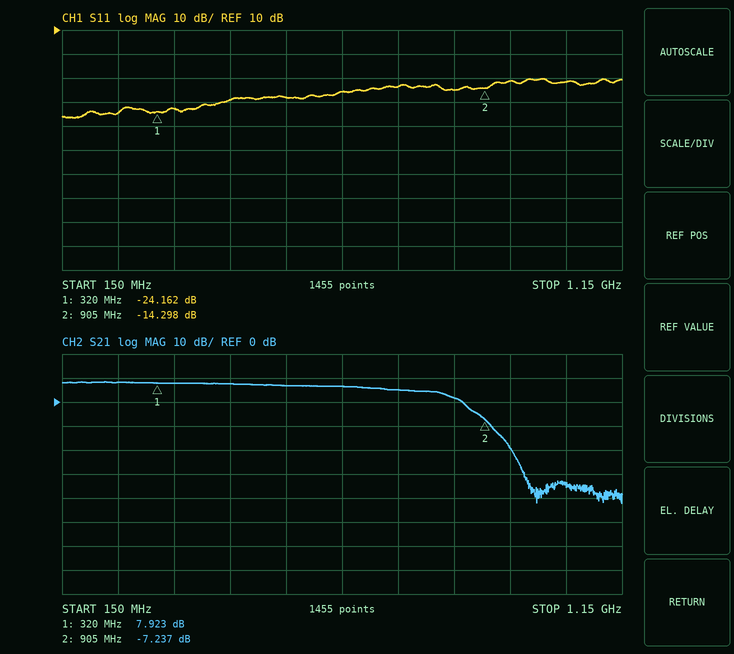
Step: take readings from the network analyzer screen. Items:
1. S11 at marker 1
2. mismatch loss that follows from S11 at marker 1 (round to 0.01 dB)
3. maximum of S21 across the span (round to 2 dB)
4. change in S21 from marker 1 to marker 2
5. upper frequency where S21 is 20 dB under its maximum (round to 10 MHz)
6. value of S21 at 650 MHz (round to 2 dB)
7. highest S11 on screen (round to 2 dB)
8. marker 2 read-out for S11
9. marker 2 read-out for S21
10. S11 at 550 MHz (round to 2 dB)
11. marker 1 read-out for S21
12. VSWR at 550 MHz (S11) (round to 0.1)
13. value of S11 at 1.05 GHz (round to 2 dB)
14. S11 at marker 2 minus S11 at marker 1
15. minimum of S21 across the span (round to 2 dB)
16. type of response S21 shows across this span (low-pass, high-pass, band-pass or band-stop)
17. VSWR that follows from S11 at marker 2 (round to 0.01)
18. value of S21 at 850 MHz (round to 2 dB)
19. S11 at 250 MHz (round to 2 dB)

-24.162 dB
0.02 dB
8 dB
-15.160 dB
920 MHz
6 dB
-10 dB
-14.298 dB
-7.237 dB
-18 dB
7.923 dB
1.3
-12 dB
9.864 dB
-42 dB
low-pass
1.48
2 dB
-24 dB
